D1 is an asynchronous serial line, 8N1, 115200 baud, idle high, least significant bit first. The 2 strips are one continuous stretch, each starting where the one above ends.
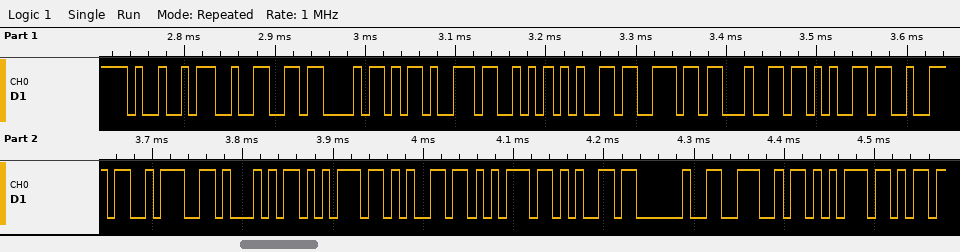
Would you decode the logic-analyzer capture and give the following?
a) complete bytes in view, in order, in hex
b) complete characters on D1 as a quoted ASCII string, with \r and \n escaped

49 32 43 2D 53 65 6E 64 65 72 3A 51 75 65 75 65 20 4E 75
"I2C-Sender:Queue Nu"
